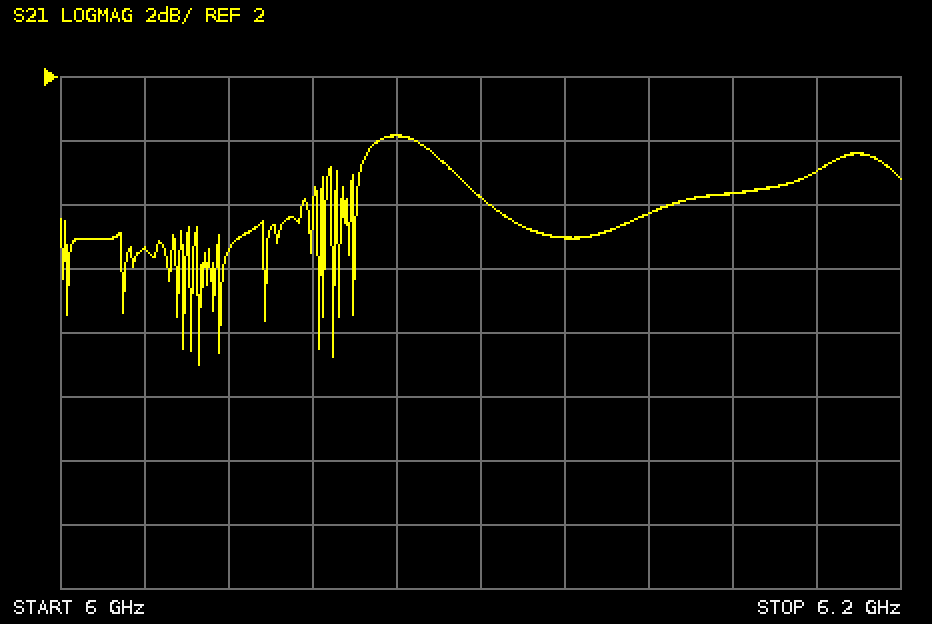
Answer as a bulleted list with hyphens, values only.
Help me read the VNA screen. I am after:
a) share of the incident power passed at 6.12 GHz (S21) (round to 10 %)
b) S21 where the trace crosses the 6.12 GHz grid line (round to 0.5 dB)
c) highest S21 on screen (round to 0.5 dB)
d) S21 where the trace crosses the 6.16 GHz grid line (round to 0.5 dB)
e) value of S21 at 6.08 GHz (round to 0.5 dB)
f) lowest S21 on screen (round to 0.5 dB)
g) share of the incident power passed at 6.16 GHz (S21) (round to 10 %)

- 50 %
- -3.0 dB
- 0.0 dB
- -1.5 dB
- 0.0 dB
- -7.0 dB
- 70 %
